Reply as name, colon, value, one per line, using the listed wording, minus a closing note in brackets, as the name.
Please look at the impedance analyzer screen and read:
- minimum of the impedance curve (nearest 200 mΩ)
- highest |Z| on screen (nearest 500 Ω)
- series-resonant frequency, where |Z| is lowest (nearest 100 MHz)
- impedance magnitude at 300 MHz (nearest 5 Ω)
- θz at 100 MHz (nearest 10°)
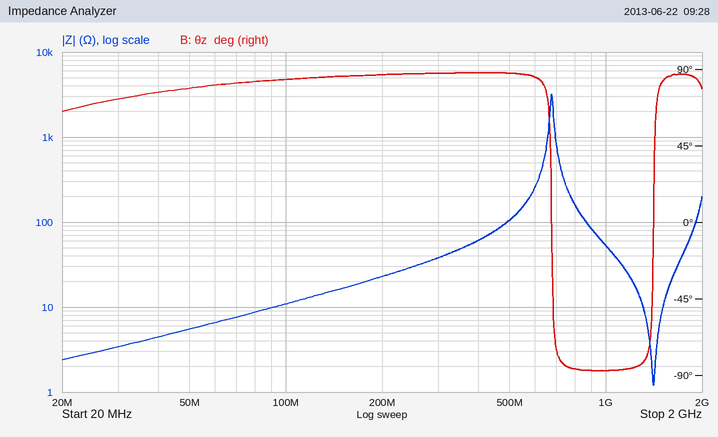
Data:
minimum of the impedance curve: 1.2 Ω
highest |Z| on screen: 3.0 kΩ
series-resonant frequency, where |Z| is lowest: 1.4 GHz
impedance magnitude at 300 MHz: 40 Ω
θz at 100 MHz: 80°
